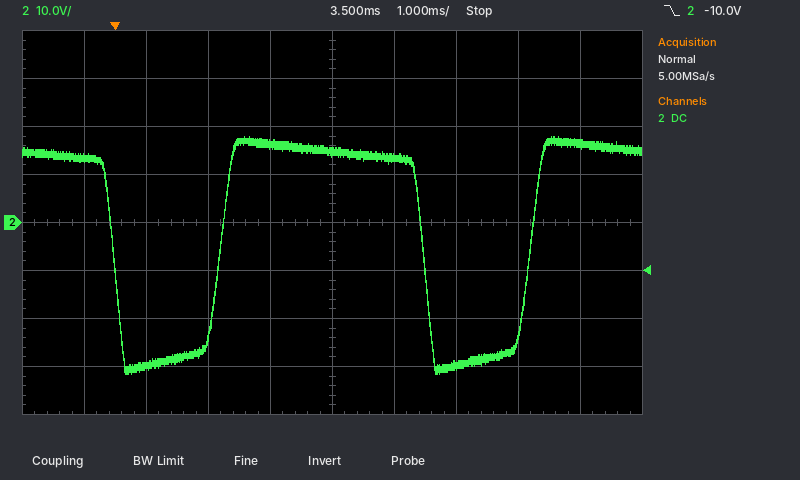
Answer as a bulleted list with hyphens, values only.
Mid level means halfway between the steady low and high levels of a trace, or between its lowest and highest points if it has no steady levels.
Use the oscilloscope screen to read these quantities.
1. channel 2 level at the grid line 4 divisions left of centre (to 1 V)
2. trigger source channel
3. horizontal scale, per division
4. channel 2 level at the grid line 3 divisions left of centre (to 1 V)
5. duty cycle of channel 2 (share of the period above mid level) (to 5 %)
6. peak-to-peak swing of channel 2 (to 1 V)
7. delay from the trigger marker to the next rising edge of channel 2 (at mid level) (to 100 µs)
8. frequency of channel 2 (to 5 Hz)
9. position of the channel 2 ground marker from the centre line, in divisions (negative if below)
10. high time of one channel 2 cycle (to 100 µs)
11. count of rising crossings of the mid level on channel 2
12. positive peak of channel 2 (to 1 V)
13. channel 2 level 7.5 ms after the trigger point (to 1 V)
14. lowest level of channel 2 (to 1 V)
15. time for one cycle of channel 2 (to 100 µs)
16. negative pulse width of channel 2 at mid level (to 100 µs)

- 13 V
- channel 2
- 1 ms
- -30 V
- 65 %
- 50 V
- 1.7 ms
- 200 Hz
- 0.0 div
- 3.3 ms
- 2
- 18 V
- 16 V
- -32 V
- 5.0 ms
- 1.7 ms
